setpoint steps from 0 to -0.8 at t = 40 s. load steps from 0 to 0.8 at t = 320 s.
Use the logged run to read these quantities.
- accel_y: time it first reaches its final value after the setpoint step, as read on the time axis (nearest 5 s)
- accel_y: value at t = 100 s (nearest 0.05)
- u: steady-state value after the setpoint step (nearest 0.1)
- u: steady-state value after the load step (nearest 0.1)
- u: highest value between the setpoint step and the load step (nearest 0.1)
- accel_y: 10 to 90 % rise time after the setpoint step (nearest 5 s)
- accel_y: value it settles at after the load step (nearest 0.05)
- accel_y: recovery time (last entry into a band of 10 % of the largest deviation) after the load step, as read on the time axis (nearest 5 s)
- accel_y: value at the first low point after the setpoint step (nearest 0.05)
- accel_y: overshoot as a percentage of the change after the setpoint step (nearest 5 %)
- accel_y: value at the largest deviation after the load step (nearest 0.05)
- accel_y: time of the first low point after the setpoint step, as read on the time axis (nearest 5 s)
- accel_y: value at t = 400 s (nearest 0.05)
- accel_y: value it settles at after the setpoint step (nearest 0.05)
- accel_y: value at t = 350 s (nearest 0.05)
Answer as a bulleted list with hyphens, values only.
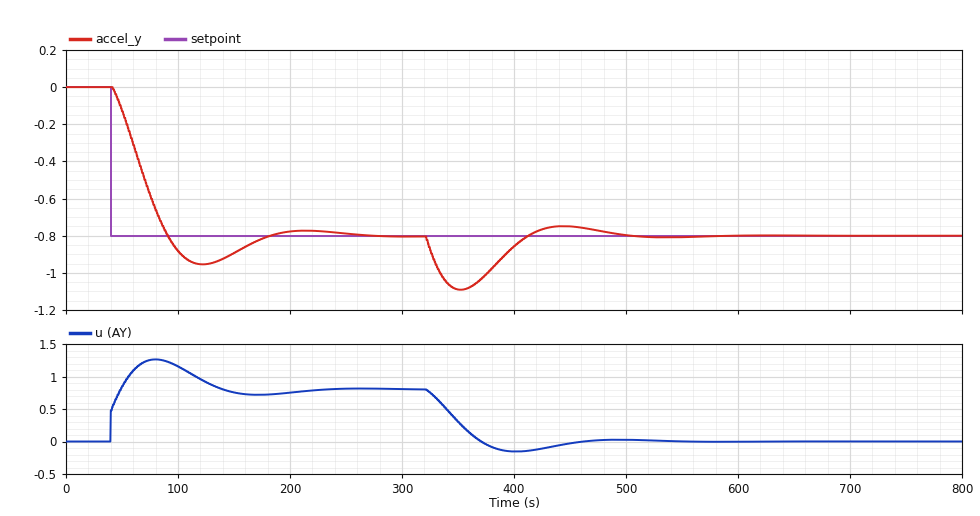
- 90 s
- -0.90
- 0.8
- 0.0
- 1.3
- 35 s
- -0.80
- 475 s
- -0.95
- 20 %
- -1.10
- 120 s
- -0.85
- -0.80
- -1.10
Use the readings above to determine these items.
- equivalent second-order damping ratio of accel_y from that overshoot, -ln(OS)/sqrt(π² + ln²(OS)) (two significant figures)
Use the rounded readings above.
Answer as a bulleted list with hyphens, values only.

- 0.46
